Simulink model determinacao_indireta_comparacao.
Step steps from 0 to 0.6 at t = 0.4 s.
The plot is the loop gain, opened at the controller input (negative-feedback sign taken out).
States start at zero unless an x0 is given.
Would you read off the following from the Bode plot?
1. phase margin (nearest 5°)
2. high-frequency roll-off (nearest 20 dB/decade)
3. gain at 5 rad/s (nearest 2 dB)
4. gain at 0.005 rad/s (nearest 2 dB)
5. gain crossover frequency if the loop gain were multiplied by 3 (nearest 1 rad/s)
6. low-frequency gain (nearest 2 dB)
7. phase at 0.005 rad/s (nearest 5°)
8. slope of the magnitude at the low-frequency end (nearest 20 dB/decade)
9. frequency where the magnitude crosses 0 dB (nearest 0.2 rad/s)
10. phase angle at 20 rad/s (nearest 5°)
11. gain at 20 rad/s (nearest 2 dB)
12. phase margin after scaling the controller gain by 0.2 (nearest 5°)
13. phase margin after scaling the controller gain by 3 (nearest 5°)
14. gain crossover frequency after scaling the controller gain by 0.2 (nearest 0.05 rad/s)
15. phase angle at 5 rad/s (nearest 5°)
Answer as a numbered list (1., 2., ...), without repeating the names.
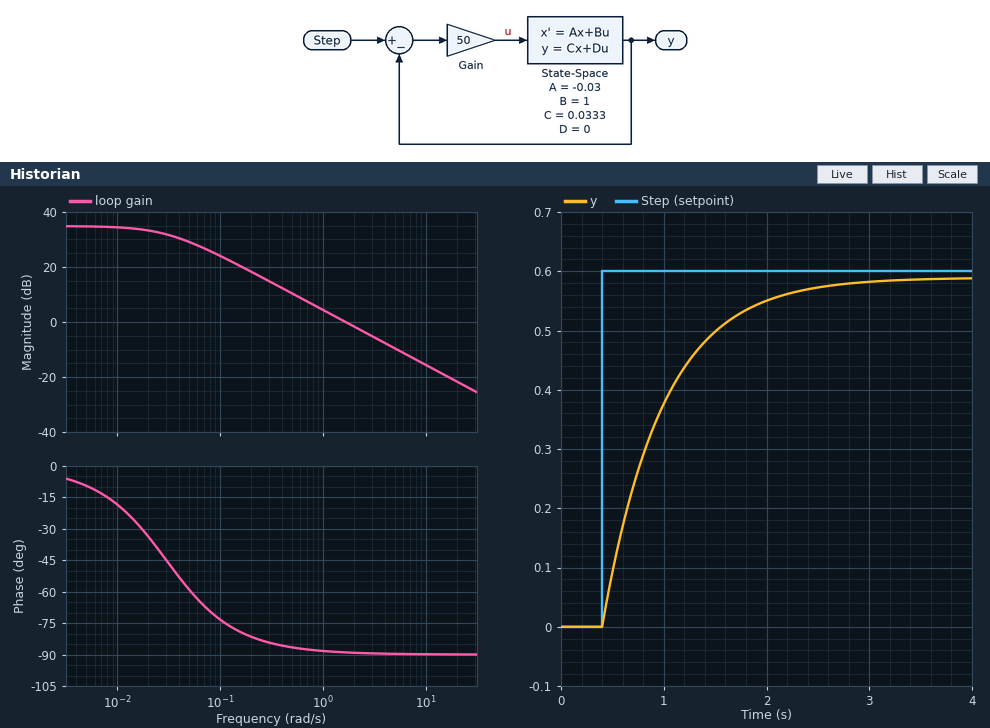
1. 90°
2. -20 dB/decade
3. -10 dB
4. 34 dB
5. 5 rad/s
6. 34 dB
7. -10°
8. 0 dB/decade
9. 1.6 rad/s
10. -90°
11. -22 dB
12. 95°
13. 90°
14. 0.35 rad/s
15. -90°
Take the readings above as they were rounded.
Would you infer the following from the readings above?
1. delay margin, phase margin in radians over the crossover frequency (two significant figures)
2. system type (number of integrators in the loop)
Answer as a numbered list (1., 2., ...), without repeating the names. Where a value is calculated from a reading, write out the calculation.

1. 90 × π / 180 / 1.6 = 0.98 s
2. 0
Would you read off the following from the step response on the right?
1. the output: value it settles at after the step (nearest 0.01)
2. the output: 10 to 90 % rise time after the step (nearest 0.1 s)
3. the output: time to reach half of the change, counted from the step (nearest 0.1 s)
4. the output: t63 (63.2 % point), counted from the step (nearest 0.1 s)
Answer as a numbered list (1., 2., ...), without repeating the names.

1. 0.59
2. 1.3 s
3. 0.4 s
4. 0.6 s
